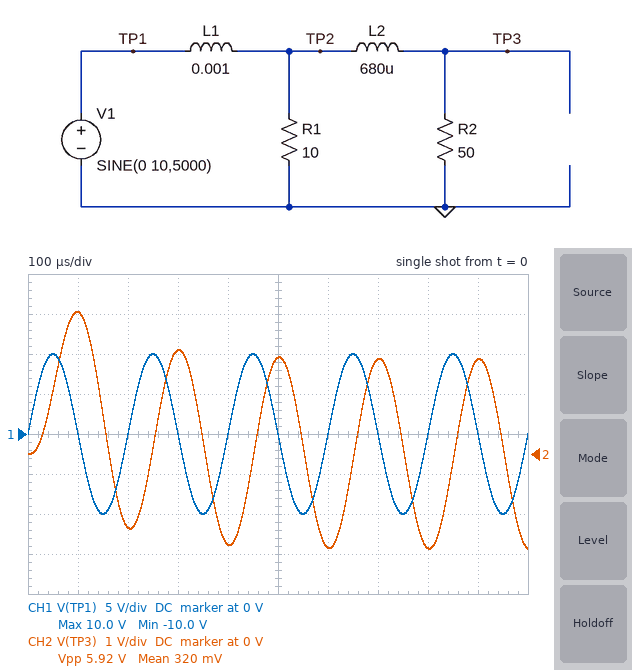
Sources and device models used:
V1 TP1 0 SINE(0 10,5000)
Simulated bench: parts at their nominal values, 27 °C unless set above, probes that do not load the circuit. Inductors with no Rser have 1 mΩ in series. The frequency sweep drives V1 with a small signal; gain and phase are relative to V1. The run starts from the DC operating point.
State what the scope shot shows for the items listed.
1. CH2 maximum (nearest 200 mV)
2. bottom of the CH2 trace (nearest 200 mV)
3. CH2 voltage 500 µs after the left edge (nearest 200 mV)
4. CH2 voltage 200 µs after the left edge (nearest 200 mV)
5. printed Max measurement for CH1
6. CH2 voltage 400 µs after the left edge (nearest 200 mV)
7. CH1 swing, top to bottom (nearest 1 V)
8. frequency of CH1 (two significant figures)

3.6 V
-2.4 V
2.4 V
-1.8 V
10.0 V
-2.2 V
20 V
5.0 kHz
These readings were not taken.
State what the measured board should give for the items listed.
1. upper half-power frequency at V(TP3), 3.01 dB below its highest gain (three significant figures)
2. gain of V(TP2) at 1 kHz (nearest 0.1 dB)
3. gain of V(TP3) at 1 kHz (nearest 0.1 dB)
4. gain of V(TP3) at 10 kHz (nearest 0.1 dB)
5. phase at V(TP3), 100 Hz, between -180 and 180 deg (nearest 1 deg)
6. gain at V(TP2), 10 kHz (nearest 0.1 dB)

1.29 kHz
-2.0 dB
-2.0 dB
-19.5 dB
-5 deg
-17.1 dB
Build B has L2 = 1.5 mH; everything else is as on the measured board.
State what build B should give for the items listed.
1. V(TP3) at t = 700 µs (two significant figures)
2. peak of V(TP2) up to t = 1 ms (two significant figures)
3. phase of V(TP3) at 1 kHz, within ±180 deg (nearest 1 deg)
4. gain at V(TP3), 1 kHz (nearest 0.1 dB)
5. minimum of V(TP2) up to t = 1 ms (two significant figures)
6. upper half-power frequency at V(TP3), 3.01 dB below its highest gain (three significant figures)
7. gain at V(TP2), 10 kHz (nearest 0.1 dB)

1.8 V
3.8 V
-47 deg
-2.2 dB
-2.7 V
1.22 kHz
-16.6 dB
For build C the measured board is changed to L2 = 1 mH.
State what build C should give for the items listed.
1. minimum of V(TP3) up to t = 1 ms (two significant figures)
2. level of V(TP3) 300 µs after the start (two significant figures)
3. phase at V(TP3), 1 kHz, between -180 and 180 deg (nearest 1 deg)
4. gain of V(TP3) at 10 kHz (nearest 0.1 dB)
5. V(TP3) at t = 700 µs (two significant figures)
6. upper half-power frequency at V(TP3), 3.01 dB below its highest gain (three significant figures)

-2.2 V
2.4 V
-44 deg
-21.0 dB
2.2 V
1.26 kHz
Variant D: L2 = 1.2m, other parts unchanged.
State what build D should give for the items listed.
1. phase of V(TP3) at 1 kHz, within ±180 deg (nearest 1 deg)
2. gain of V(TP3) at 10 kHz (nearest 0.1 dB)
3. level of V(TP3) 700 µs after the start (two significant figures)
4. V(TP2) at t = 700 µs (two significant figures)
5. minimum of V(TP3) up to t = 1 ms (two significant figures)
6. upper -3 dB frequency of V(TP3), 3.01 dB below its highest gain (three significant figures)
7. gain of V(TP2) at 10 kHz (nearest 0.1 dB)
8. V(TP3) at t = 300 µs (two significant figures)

-45 deg
-21.9 dB
2.0 V
2.5 V
-2.1 V
1.25 kHz
-16.7 dB
2.3 V
